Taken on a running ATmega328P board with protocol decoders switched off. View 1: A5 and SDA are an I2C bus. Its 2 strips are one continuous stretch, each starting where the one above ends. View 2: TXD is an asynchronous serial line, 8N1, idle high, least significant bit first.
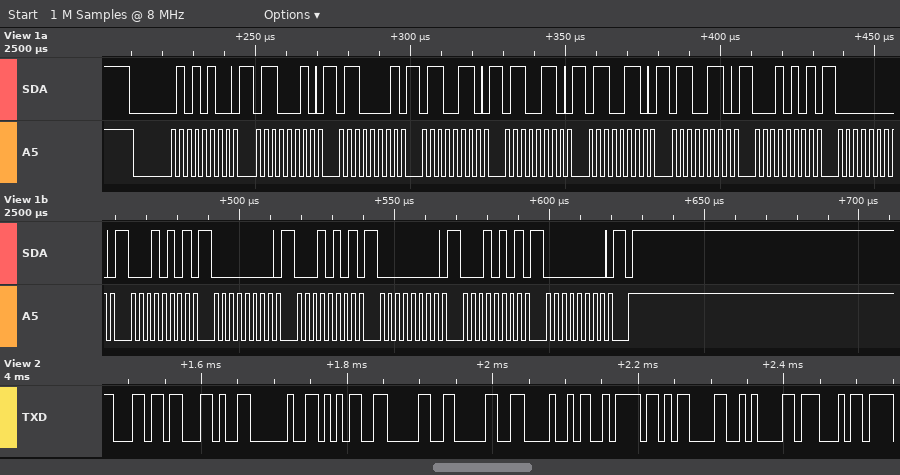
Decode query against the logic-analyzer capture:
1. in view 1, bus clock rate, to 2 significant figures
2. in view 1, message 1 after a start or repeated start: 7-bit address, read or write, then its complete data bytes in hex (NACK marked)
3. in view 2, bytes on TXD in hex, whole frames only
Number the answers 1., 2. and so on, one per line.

1. 400 kHz
2. 0x2A write: 62 61 66 66 66 66 15 00 15 00 15 00 15 00
3. 6C 2C 20 35 30 30 48 7A 0D 0A 47
